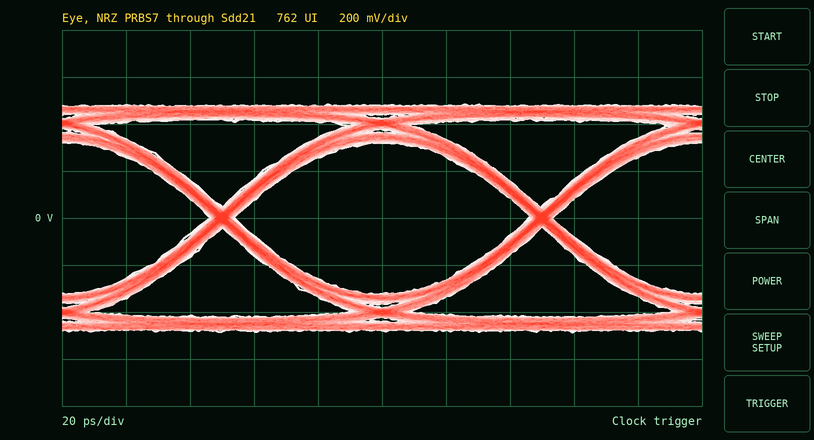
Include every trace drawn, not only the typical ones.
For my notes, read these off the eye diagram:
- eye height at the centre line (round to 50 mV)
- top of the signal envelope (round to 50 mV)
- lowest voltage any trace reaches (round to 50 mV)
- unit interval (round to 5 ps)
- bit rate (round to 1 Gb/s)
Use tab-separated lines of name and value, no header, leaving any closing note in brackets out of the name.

eye height at the centre line	650 mV
top of the signal envelope	500 mV
lowest voltage any trace reaches	-500 mV
unit interval	100 ps
bit rate	10 Gb/s
